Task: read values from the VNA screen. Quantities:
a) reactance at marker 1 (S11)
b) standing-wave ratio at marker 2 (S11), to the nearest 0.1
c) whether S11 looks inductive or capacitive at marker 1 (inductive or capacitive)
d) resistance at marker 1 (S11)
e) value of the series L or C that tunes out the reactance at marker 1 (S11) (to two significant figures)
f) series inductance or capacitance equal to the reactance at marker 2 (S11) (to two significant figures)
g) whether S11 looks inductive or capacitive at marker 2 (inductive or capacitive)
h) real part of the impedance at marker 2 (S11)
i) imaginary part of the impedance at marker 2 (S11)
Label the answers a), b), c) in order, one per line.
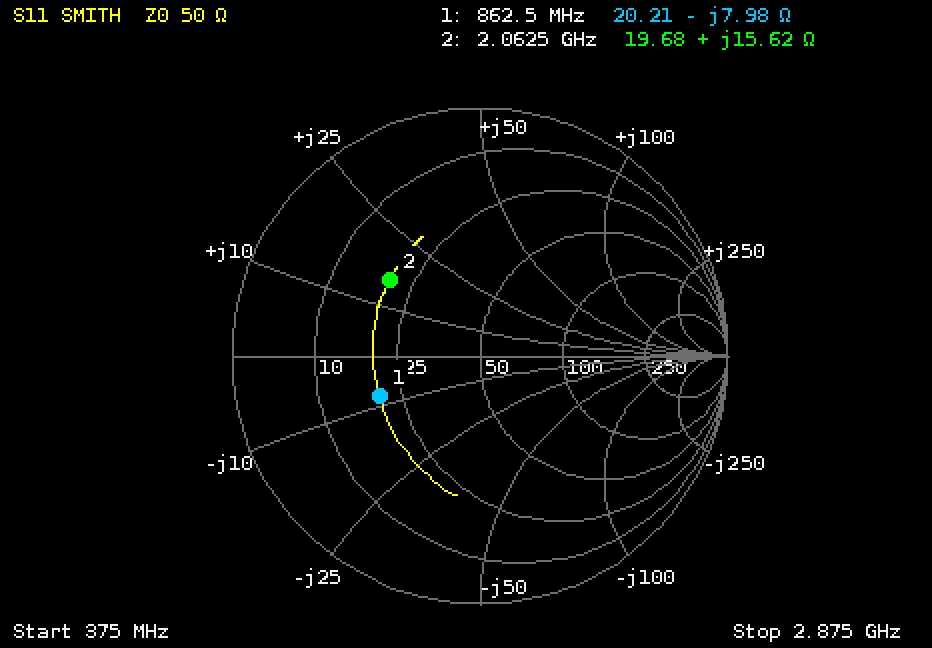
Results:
a) -7.98 Ω
b) 2.8
c) capacitive
d) 20.21 Ω
e) 1.5 nH
f) 1.2 nH
g) inductive
h) 19.68 Ω
i) +15.62 Ω
